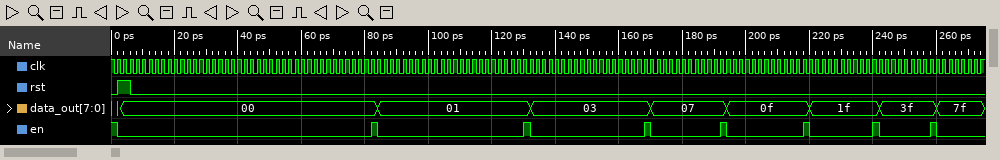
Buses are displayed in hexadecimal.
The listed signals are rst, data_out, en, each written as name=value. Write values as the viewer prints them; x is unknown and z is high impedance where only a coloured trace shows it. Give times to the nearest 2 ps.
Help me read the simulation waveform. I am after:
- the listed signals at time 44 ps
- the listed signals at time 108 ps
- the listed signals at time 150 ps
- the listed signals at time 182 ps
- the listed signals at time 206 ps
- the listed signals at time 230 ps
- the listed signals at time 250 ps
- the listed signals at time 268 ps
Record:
rst=0, data_out=00, en=0
rst=0, data_out=01, en=0
rst=0, data_out=03, en=0
rst=0, data_out=07, en=0
rst=0, data_out=0f, en=0
rst=0, data_out=1f, en=0
rst=0, data_out=3f, en=0
rst=0, data_out=7f, en=0
